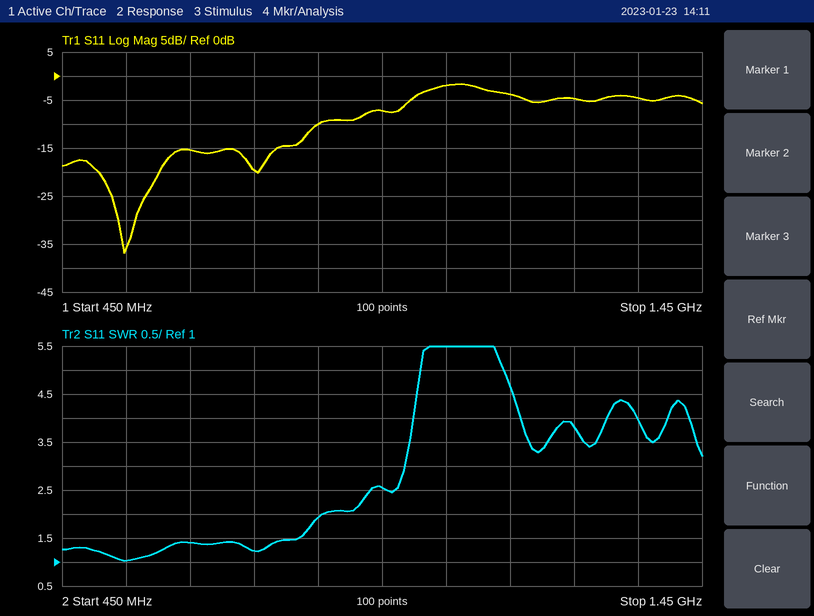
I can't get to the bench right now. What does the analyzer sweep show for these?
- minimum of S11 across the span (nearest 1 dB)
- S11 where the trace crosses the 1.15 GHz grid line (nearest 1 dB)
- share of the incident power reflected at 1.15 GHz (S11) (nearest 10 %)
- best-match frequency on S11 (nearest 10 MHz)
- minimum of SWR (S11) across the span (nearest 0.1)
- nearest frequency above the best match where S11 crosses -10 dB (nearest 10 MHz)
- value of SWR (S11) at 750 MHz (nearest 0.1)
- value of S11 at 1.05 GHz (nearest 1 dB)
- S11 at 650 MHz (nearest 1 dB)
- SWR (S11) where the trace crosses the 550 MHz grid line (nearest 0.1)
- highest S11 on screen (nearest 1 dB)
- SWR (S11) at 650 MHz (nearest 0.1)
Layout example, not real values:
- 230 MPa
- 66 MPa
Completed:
- -37 dB
- -4 dB
- 40 %
- 550 MHz
- 1.0
- 850 MHz
- 1.2
- -2 dB
- -15 dB
- 1.0
- -2 dB
- 1.4
